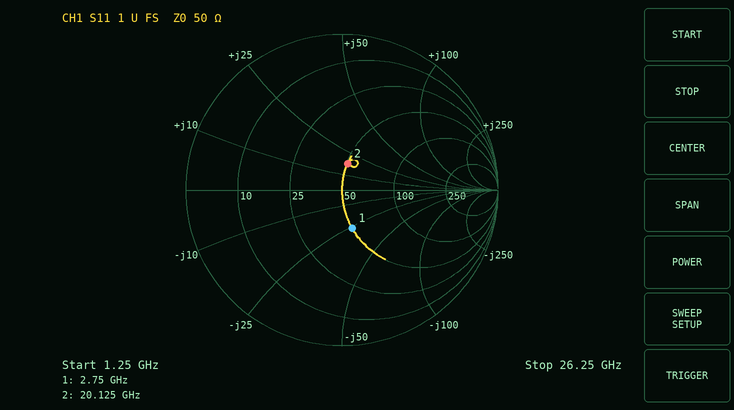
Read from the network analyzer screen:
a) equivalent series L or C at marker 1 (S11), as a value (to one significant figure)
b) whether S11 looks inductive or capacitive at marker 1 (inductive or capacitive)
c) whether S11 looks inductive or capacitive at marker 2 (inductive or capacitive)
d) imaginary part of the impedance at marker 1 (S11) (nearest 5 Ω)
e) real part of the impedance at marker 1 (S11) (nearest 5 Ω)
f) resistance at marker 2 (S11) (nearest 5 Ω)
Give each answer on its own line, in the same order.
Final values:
2 pF
capacitive
inductive
-25 Ω
50 Ω
50 Ω
